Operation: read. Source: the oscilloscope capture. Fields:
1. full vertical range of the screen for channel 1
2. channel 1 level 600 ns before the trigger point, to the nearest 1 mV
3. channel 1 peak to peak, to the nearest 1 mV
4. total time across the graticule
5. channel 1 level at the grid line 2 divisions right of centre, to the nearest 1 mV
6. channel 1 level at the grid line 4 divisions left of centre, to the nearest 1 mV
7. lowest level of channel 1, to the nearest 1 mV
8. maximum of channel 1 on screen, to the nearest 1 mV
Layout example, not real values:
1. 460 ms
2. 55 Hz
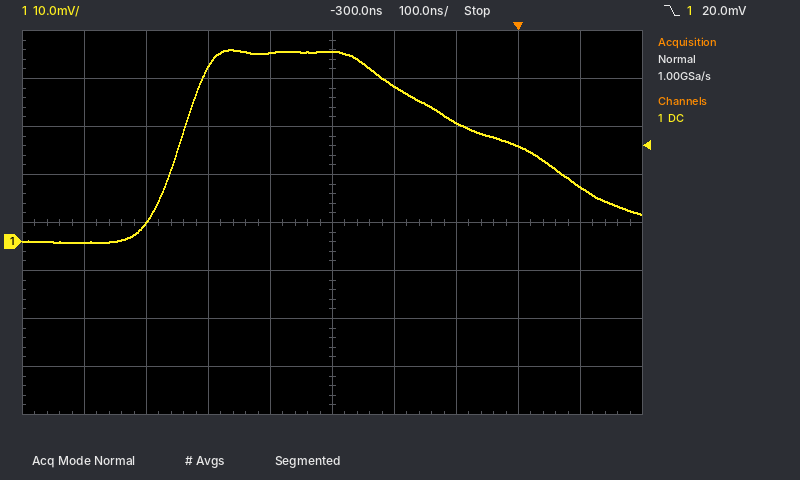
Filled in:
1. 80 mV
2. 4 mV
3. 40 mV
4. 1 µs
5. 25 mV
6. 0 mV
7. 0 mV
8. 40 mV
